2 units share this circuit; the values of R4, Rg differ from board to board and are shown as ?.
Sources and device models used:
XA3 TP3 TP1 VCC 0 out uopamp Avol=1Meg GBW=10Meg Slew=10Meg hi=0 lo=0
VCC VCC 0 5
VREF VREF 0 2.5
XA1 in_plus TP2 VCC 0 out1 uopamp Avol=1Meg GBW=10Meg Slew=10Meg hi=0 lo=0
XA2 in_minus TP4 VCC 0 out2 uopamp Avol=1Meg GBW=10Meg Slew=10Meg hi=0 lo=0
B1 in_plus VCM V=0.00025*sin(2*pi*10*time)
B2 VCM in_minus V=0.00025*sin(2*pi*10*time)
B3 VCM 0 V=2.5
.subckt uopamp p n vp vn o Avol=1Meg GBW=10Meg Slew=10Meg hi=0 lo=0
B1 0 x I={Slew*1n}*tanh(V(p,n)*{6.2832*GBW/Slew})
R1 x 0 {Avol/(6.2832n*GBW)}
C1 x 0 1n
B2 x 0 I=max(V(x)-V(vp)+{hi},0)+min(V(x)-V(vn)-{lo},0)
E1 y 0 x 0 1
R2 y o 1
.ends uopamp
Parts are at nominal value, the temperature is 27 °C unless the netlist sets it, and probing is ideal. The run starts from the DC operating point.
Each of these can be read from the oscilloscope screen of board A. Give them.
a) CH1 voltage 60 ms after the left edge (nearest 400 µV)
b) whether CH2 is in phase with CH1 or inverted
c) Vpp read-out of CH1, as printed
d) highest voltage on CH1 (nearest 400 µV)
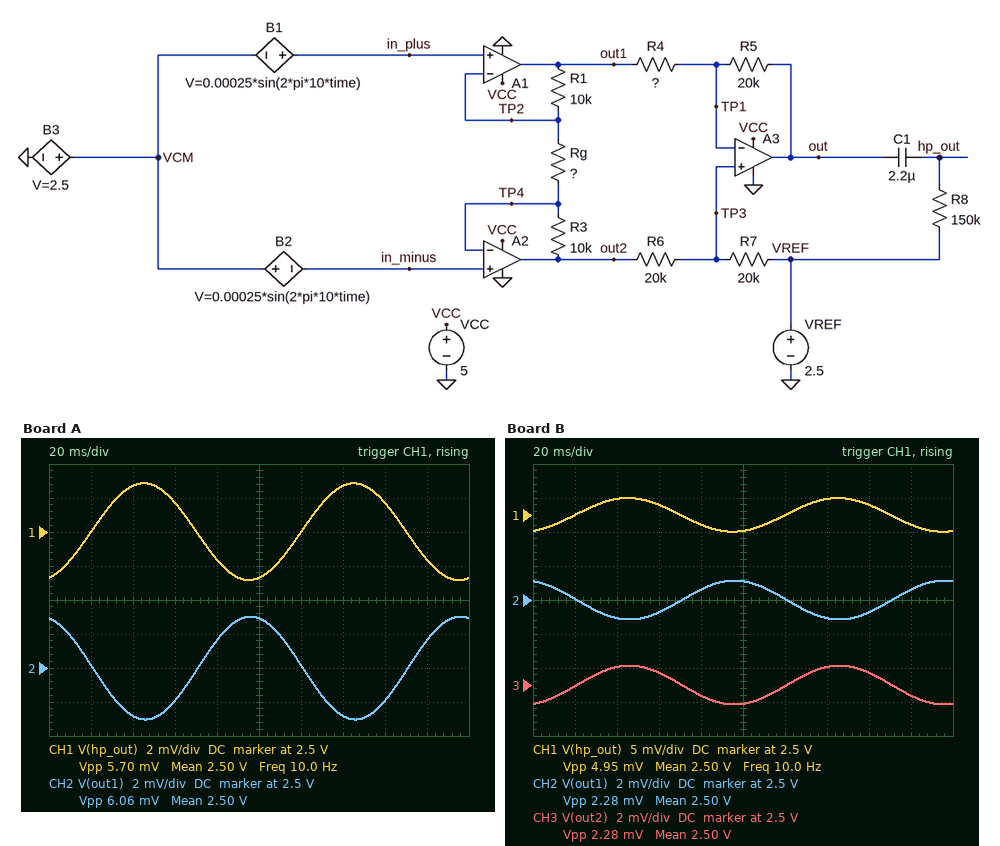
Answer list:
2.5016 V
inverted
5.70 mV
2.5028 V
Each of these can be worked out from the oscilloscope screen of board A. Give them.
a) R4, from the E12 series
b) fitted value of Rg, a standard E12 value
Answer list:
68 kΩ
1.8 kΩ
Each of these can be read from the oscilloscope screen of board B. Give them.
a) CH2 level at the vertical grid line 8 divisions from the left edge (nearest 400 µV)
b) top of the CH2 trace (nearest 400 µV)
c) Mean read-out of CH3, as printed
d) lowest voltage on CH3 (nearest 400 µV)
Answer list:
2.4992 V
2.5012 V
2.50 V
2.4988 V
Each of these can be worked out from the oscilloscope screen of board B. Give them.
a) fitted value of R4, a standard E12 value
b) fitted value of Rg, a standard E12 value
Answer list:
18 kΩ
5.6 kΩ
